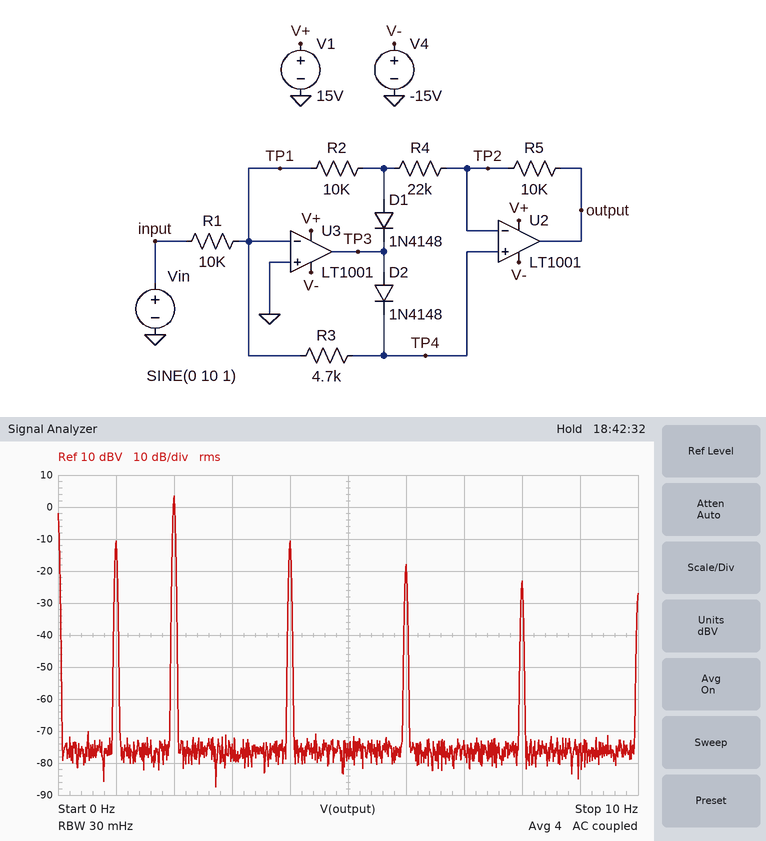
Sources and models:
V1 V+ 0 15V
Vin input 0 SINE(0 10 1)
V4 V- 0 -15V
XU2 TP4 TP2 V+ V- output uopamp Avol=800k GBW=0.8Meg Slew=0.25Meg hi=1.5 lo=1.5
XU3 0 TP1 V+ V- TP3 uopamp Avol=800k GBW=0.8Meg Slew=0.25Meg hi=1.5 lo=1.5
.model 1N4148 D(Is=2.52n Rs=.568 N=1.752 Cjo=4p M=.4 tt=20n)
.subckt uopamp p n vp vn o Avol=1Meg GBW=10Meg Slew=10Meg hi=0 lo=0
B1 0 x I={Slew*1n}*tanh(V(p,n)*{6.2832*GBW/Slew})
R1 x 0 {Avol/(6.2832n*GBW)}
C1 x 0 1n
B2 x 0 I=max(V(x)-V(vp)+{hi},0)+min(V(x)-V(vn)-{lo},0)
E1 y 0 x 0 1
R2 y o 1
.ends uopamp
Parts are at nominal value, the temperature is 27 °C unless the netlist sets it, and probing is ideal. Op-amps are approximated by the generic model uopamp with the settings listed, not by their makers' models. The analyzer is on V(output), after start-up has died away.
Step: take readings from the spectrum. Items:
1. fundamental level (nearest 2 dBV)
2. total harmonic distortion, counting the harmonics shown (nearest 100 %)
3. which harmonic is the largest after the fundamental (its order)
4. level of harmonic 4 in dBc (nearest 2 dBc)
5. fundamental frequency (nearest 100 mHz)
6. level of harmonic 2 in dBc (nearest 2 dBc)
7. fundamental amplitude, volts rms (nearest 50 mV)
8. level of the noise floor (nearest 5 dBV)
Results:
-10 dBV
500 %
2
0 dBc
1.0 Hz
14 dBc
300 mV
-75 dBV
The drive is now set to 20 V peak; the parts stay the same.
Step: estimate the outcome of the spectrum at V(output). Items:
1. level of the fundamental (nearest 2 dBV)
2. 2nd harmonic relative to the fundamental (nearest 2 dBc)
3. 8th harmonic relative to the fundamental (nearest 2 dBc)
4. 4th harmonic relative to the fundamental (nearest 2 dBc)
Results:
-18 dBV
28 dBc
2 dBc
12 dBc
